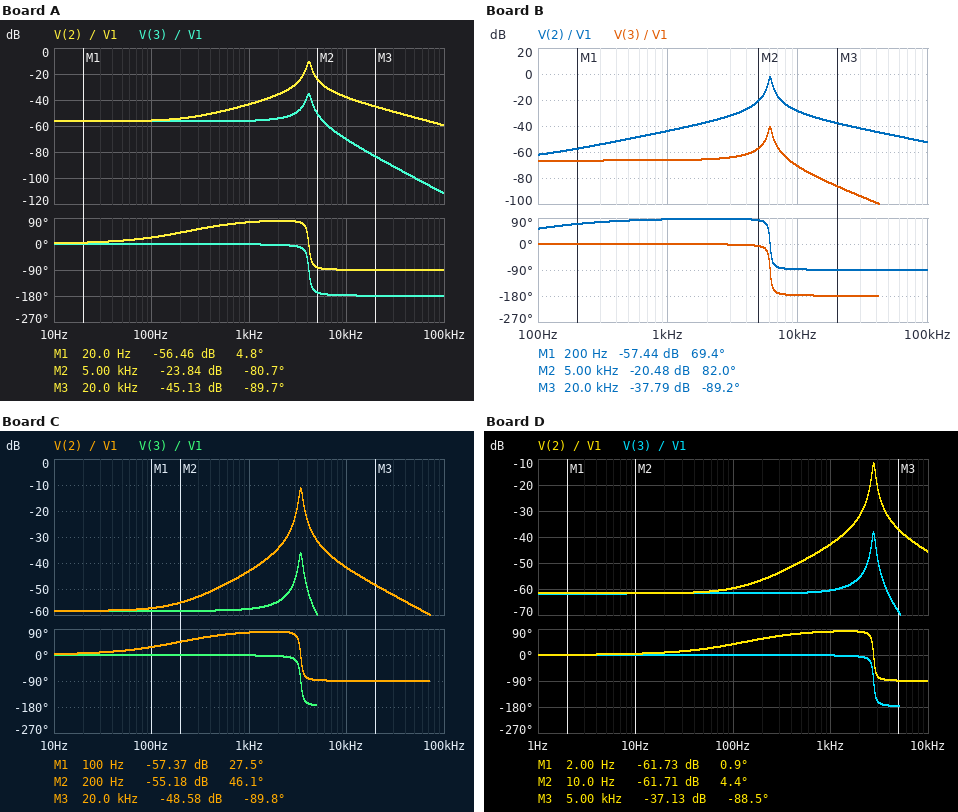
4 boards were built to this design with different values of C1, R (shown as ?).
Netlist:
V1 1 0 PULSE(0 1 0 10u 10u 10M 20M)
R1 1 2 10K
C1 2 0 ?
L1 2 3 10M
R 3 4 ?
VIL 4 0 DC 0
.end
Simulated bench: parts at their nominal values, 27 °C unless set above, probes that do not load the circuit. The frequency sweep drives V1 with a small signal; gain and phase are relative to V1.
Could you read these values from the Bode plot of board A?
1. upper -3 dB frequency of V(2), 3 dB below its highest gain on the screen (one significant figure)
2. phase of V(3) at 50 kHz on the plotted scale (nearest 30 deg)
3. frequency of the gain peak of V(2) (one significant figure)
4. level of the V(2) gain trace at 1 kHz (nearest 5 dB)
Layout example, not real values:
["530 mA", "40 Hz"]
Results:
["4 kHz", "-180 deg", "4 kHz", "-45 dB"]
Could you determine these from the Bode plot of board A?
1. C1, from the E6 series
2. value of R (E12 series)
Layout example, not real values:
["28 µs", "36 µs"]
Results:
["150 nF", "15 Ω"]
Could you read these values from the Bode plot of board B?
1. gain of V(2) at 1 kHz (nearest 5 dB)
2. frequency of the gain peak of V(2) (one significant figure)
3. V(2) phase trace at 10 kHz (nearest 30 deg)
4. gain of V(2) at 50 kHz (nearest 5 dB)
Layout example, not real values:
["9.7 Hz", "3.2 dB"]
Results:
["-45 dB", "6 kHz", "-90 deg", "-45 dB"]
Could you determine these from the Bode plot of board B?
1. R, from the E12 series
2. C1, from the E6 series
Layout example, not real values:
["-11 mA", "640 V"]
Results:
["4.7 Ω", "68 nF"]
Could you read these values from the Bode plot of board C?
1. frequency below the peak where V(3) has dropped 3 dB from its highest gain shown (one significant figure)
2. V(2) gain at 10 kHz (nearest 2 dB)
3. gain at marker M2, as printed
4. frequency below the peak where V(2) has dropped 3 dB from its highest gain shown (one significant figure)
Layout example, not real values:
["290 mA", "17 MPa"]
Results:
["3 kHz", "-42 dB", "-55.18 dB", "3 kHz"]
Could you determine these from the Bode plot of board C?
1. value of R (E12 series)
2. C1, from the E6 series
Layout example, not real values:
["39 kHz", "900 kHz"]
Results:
["12 Ω", "220 nF"]
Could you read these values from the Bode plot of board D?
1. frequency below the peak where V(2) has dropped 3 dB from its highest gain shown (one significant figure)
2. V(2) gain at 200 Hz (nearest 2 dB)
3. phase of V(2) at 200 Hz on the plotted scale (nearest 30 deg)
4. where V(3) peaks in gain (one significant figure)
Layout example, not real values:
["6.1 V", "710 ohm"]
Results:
["3 kHz", "-56 dB", "60 deg", "3 kHz"]
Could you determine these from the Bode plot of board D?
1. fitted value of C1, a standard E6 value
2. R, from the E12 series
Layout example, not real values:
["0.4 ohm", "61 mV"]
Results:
["330 nF", "8.2 Ω"]
